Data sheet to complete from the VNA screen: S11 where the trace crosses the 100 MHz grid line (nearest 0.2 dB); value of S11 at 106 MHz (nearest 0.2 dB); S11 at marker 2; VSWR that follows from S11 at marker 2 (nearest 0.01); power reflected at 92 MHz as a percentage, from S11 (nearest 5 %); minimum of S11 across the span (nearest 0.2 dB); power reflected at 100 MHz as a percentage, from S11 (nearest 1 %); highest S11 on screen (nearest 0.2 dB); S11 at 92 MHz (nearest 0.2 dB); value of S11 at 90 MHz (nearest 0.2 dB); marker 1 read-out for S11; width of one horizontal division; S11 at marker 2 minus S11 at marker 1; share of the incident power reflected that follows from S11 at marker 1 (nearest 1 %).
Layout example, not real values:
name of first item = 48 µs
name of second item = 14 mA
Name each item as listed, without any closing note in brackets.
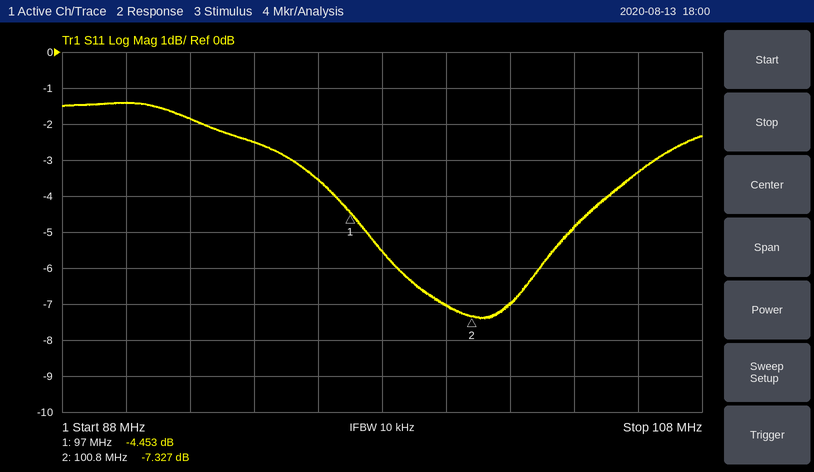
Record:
S11 where the trace crosses the 100 MHz grid line = -7.0 dB
value of S11 at 106 MHz = -3.4 dB
S11 at marker 2 = -7.327 dB
VSWR that follows from S11 at marker 2 = 2.51
power reflected at 92 MHz as a percentage, from S11 = 65 %
minimum of S11 across the span = -7.4 dB
power reflected at 100 MHz as a percentage, from S11 = 20 %
highest S11 on screen = -1.4 dB
S11 at 92 MHz = -1.8 dB
value of S11 at 90 MHz = -1.4 dB
marker 1 read-out for S11 = -4.453 dB
width of one horizontal division = 2 MHz
S11 at marker 2 minus S11 at marker 1 = -2.874 dB
share of the incident power reflected that follows from S11 at marker 1 = 36 %
